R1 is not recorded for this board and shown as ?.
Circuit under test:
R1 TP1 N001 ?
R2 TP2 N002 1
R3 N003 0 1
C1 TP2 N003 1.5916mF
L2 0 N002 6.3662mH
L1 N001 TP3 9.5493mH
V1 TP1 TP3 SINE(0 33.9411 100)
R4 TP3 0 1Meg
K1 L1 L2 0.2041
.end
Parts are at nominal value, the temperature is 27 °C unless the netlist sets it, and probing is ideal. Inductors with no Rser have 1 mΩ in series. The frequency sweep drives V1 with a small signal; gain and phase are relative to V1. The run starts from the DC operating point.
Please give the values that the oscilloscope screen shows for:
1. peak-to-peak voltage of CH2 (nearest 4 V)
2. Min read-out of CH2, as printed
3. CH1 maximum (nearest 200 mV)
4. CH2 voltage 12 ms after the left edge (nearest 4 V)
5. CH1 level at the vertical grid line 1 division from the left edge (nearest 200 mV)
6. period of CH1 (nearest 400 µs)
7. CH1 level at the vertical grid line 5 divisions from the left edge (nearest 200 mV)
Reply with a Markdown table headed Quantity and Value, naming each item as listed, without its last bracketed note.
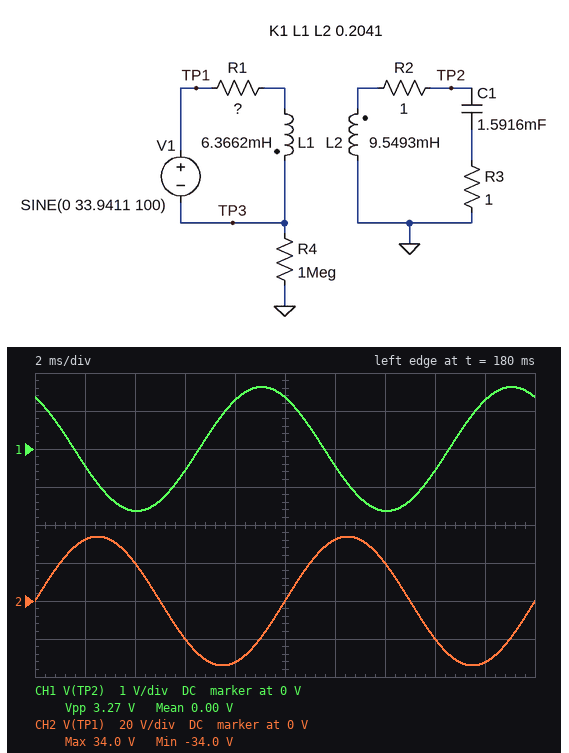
| Quantity | Value |
|---|---|
| peak-to-peak voltage of CH2 | 68 V |
| Min read-out of CH2, as printed | -34.0 V |
| CH1 maximum | 1.6 V |
| CH2 voltage 12 ms after the left edge | 32 V |
| CH1 level at the vertical grid line 1 division from the left edge | -400 mV |
| period of CH1 | 10.0 ms |
| CH1 level at the vertical grid line 5 divisions from the left edge | 1.4 V |
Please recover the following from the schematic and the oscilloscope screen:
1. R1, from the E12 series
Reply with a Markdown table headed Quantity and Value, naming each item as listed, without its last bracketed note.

| Quantity | Value |
|---|---|
| R1, from the E12 series | 5.6 Ω |
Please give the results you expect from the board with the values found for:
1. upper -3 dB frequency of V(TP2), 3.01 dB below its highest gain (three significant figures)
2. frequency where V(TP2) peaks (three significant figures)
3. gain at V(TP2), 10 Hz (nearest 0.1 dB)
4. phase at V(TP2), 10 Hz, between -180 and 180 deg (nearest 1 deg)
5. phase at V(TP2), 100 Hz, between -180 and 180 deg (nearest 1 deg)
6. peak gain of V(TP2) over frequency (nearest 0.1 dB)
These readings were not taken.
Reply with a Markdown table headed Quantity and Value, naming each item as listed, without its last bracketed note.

| Quantity | Value |
|---|---|
| upper -3 dB frequency of V(TP2), 3.01 dB below its highest gain | 81.0 Hz |
| frequency where V(TP2) peaks | 49.6 Hz |
| gain at V(TP2), 10 Hz | -34.8 dB |
| phase at V(TP2), 10 Hz, between -180 and 180 deg | -102 deg |
| phase at V(TP2), 100 Hz, between -180 and 180 deg | 124 deg |
| peak gain of V(TP2) over frequency | -21.3 dB |
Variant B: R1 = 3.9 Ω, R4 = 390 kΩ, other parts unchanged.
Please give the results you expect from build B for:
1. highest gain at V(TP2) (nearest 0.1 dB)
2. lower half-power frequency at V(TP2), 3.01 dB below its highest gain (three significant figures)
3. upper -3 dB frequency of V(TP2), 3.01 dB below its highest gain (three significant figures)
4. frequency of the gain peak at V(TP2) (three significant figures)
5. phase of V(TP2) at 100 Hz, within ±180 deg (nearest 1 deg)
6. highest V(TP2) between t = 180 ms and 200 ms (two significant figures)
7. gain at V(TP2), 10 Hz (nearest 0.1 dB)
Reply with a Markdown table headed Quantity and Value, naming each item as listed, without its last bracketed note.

| Quantity | Value |
|---|---|
| highest gain at V(TP2) | -19.0 dB |
| lower half-power frequency at V(TP2), 3.01 dB below its highest gain | 28.7 Hz |
| upper -3 dB frequency of V(TP2), 3.01 dB below its highest gain | 76.2 Hz |
| frequency of the gain peak at V(TP2) | 47.9 Hz |
| phase of V(TP2) at 100 Hz, within ±180 deg | 114 deg |
| highest V(TP2) between t = 180 ms and 200 ms | 1.9 V |
| gain at V(TP2), 10 Hz | -31.7 dB |
